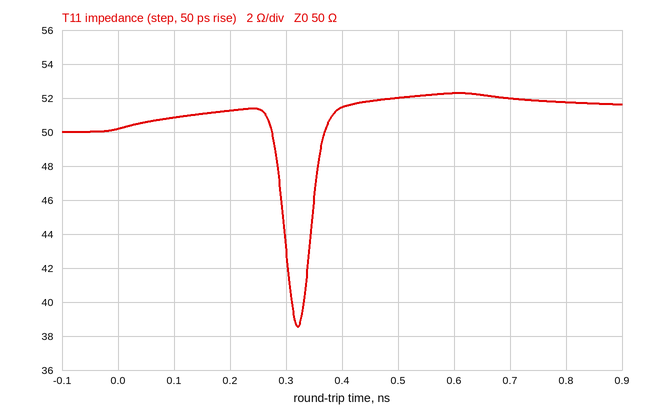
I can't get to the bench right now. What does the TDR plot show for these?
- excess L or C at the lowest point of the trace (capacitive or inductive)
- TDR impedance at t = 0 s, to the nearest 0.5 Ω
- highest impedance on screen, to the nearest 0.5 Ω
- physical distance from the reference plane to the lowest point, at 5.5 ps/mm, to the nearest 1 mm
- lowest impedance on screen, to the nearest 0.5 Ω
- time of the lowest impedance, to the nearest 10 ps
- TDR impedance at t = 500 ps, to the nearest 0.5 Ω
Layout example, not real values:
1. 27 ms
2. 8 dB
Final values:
1. capacitive
2. 50.0 Ω
3. 52.5 Ω
4. 29 mm
5. 38.5 Ω
6. 320 ps
7. 52.0 Ω
